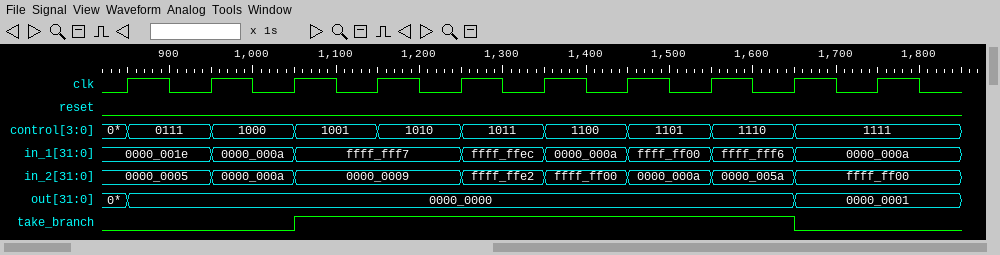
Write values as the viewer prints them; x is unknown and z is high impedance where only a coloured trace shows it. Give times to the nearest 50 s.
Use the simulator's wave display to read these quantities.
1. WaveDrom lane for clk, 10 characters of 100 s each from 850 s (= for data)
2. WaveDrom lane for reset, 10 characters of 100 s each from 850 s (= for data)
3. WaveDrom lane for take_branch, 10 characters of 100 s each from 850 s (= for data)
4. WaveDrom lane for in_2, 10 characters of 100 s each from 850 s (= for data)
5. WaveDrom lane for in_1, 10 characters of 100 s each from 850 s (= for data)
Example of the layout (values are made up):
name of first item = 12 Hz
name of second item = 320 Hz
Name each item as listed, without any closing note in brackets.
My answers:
WaveDrom lane for clk, 10 characters of 100 s each from 850 s = {name: 'clk', wave: 'p.........'}
WaveDrom lane for reset, 10 characters of 100 s each from 850 s = {name: 'reset', wave: '0.........'}
WaveDrom lane for take_branch, 10 characters of 100 s each from 850 s = {name: 'take_branch', wave: '0.1.....0.'}
WaveDrom lane for in_2, 10 characters of 100 s each from 850 s = {name: 'in_2', wave: '===.=====.', data: '0000_0005 0000_000a 0000_0009 ffff_ffe2 ffff_ff00 0000_000a 0000_005a ffff_ff00'}
WaveDrom lane for in_1, 10 characters of 100 s each from 850 s = {name: 'in_1', wave: '===.=====.', data: '0000_001e 0000_000a ffff_fff7 ffff_ffec 0000_000a ffff_ff00 ffff_fff6 0000_000a'}
